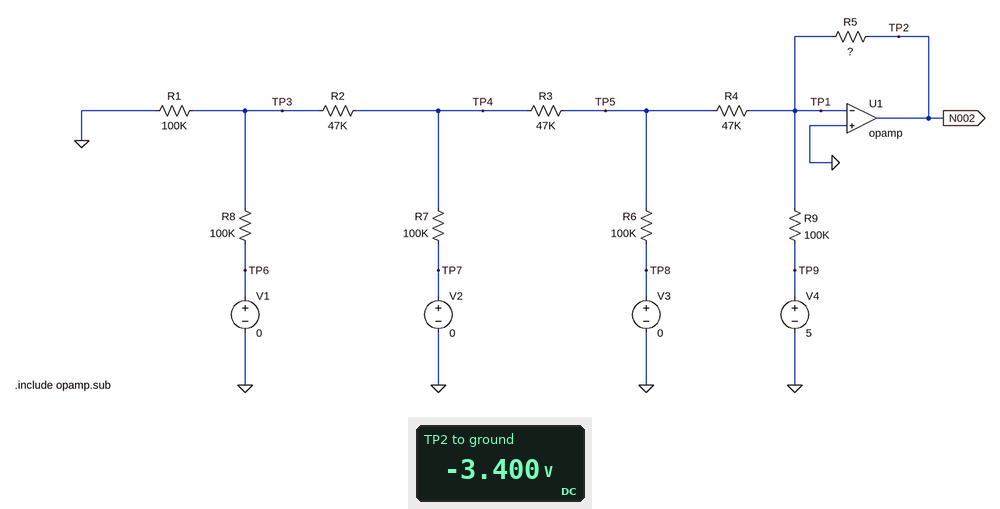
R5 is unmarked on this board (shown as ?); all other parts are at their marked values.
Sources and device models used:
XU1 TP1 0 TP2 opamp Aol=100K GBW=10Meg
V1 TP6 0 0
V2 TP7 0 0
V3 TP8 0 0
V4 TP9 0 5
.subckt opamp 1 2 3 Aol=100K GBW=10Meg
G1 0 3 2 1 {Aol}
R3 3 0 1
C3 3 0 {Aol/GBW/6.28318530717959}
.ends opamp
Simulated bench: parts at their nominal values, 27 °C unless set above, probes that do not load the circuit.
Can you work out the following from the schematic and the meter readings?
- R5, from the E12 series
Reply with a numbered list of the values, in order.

1. 68 kΩ
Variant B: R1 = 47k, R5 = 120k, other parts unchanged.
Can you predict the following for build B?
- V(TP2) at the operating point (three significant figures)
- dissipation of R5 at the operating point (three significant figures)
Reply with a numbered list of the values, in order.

1. -6.00 V
2. 300 µW
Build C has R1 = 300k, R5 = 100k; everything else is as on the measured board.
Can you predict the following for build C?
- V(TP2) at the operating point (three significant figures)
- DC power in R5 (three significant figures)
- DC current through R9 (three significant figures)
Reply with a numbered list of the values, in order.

1. -5.00 V
2. 250 µW
3. 50.0 µA
